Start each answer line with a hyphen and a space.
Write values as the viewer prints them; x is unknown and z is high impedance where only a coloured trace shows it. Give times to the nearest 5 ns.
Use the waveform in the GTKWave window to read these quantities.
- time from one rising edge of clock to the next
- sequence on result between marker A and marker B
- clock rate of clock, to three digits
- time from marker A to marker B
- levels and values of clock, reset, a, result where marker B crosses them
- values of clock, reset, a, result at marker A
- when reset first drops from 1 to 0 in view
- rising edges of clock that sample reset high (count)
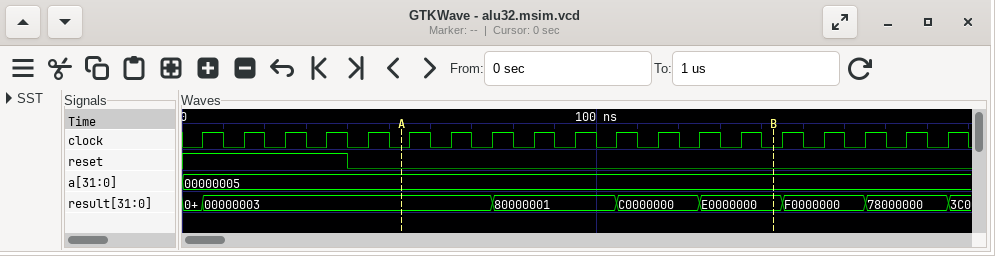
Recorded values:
- 10 ns
- 00000003, 80000001, C0000000, E0000000
- 100 MHz
- 90 ns
- clock=0, reset=0, a=00000005, result=E0000000
- clock=0, reset=0, a=00000005, result=00000003
- 40 ns
- 4
